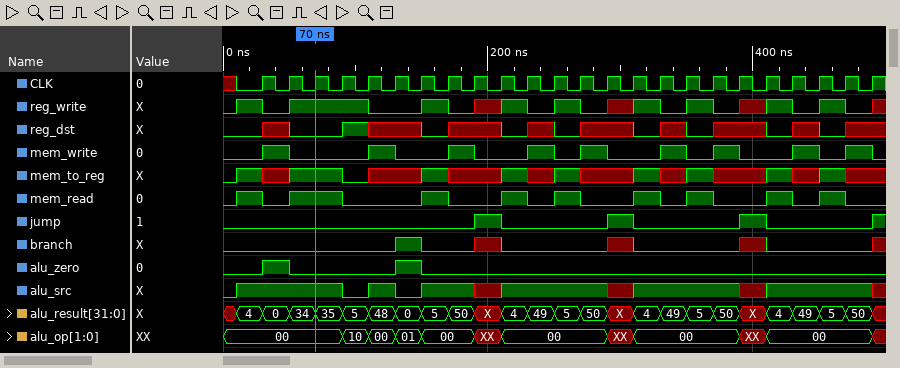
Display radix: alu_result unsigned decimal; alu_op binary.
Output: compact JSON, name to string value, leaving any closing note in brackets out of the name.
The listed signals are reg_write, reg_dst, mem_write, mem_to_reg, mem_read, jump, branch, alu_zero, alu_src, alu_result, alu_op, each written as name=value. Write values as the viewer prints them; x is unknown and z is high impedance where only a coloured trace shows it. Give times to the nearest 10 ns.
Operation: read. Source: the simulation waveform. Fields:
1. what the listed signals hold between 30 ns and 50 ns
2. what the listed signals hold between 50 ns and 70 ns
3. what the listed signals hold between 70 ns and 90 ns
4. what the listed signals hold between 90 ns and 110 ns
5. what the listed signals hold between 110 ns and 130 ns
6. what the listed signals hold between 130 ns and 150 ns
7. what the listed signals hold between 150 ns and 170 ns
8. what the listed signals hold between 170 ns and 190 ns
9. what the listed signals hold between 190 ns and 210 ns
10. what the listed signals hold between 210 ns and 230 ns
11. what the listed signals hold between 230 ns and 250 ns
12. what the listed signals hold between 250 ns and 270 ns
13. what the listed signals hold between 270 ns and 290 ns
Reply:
{"what the listed signals hold between 30 ns and 50 ns": "reg_write=0, reg_dst=x, mem_write=1, mem_to_reg=x, mem_read=0, jump=0, branch=0, alu_zero=1, alu_src=1, alu_result=0, alu_op=00", "what the listed signals hold between 50 ns and 70 ns": "reg_write=1, reg_dst=0, mem_write=0, mem_to_reg=1, mem_read=1, jump=0, branch=0, alu_zero=0, alu_src=1, alu_result=34, alu_op=00", "what the listed signals hold between 70 ns and 90 ns": "reg_write=1, reg_dst=0, mem_write=0, mem_to_reg=1, mem_read=1, jump=0, branch=0, alu_zero=0, alu_src=1, alu_result=35, alu_op=00", "what the listed signals hold between 90 ns and 110 ns": "reg_write=1, reg_dst=1, mem_write=0, mem_to_reg=0, mem_read=0, jump=0, branch=0, alu_zero=0, alu_src=0, alu_result=5, alu_op=10", "what the listed signals hold between 110 ns and 130 ns": "reg_write=0, reg_dst=x, mem_write=1, mem_to_reg=x, mem_read=0, jump=0, branch=0, alu_zero=0, alu_src=1, alu_result=48, alu_op=00", "what the listed signals hold between 130 ns and 150 ns": "reg_write=0, reg_dst=x, mem_write=0, mem_to_reg=x, mem_read=0, jump=0, branch=1, alu_zero=1, alu_src=0, alu_result=0, alu_op=01", "what the listed signals hold between 150 ns and 170 ns": "reg_write=1, reg_dst=0, mem_write=0, mem_to_reg=1, mem_read=1, jump=0, branch=0, alu_zero=0, alu_src=1, alu_result=5, alu_op=00", "what the listed signals hold between 170 ns and 190 ns": "reg_write=0, reg_dst=x, mem_write=1, mem_to_reg=x, mem_read=0, jump=0, branch=0, alu_zero=0, alu_src=1, alu_result=50, alu_op=00", "what the listed signals hold between 190 ns and 210 ns": "reg_write=x, reg_dst=x, mem_write=0, mem_to_reg=x, mem_read=0, jump=1, branch=x, alu_zero=0, alu_src=x, alu_result=X, alu_op=XX", "what the listed signals hold between 210 ns and 230 ns": "reg_write=1, reg_dst=0, mem_write=0, mem_to_reg=1, mem_read=1, jump=0, branch=0, alu_zero=0, alu_src=1, alu_result=4, alu_op=00", "what the listed signals hold between 230 ns and 250 ns": "reg_write=0, reg_dst=x, mem_write=1, mem_to_reg=x, mem_read=0, jump=0, branch=0, alu_zero=0, alu_src=1, alu_result=49, alu_op=00", "what the listed signals hold between 250 ns and 270 ns": "reg_write=1, reg_dst=0, mem_write=0, mem_to_reg=1, mem_read=1, jump=0, branch=0, alu_zero=0, alu_src=1, alu_result=5, alu_op=00", "what the listed signals hold between 270 ns and 290 ns": "reg_write=0, reg_dst=x, mem_write=1, mem_to_reg=x, mem_read=0, jump=0, branch=0, alu_zero=0, alu_src=1, alu_result=50, alu_op=00"}
